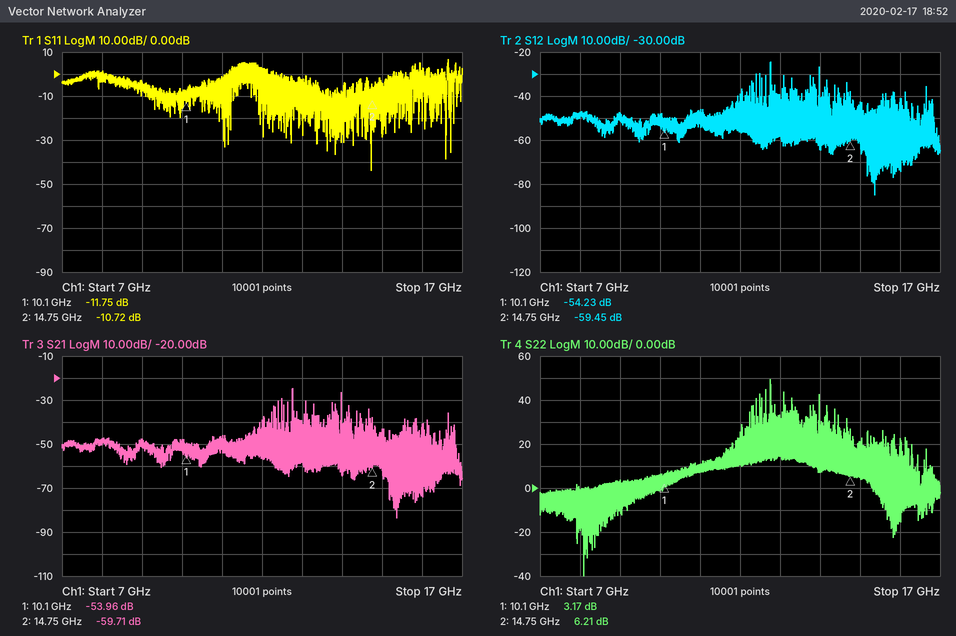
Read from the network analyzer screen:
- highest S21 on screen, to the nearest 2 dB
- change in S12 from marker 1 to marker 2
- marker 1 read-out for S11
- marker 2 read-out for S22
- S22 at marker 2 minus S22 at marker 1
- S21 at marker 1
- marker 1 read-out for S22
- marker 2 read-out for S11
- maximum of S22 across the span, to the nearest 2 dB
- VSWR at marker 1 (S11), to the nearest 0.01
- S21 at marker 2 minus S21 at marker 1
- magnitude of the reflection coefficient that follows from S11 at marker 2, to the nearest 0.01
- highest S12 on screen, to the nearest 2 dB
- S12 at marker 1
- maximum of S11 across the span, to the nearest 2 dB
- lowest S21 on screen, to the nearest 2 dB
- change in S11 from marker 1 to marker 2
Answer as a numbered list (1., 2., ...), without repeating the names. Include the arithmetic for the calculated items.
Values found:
1. -24 dB
2. -59.45 − (-54.23) = -5.22 dB
3. -11.75 dB
4. 6.21 dB
5. 6.21 − (3.17) = 3.04 dB
6. -53.96 dB
7. 3.17 dB
8. -10.72 dB
9. 50 dB
10. (1 + 0.2585)/(1 − 0.2585) ≈ 1.70
11. -59.71 − (-53.96) = -5.75 dB
12. 10^(-10.72/20) ≈ 0.29
13. -24 dB
14. -54.23 dB
15. 6 dB
16. -84 dB
17. -10.72 − (-11.75) = 1.03 dB
